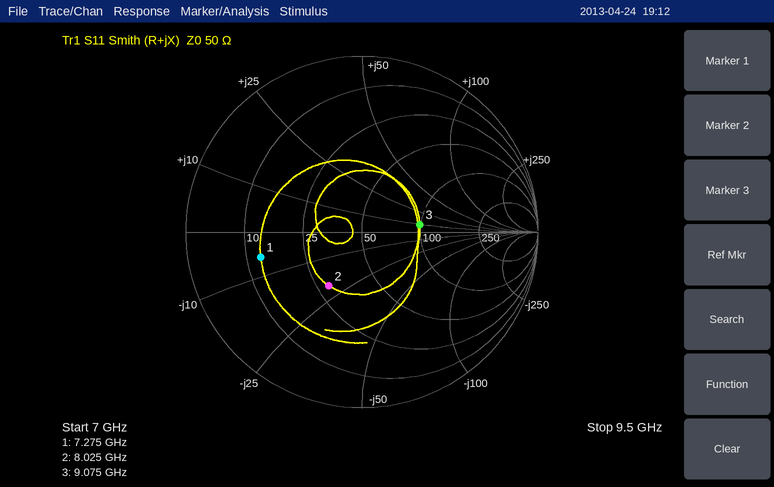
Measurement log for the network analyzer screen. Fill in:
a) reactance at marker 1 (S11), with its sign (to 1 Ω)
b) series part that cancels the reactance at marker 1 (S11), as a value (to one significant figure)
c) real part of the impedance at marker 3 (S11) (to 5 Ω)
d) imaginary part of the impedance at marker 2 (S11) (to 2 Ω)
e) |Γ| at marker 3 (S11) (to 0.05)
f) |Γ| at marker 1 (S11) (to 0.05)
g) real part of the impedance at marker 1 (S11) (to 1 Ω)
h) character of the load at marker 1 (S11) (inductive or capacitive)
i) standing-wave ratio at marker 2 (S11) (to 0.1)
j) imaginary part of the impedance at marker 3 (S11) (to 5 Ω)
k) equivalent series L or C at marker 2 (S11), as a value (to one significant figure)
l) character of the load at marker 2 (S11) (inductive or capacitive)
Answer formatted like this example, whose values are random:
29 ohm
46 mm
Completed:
-6 Ω
100 pH
100 Ω
-20 Ω
0.35
0.60
13 Ω
capacitive
2.1
+10 Ω
1.0 pF
capacitive
